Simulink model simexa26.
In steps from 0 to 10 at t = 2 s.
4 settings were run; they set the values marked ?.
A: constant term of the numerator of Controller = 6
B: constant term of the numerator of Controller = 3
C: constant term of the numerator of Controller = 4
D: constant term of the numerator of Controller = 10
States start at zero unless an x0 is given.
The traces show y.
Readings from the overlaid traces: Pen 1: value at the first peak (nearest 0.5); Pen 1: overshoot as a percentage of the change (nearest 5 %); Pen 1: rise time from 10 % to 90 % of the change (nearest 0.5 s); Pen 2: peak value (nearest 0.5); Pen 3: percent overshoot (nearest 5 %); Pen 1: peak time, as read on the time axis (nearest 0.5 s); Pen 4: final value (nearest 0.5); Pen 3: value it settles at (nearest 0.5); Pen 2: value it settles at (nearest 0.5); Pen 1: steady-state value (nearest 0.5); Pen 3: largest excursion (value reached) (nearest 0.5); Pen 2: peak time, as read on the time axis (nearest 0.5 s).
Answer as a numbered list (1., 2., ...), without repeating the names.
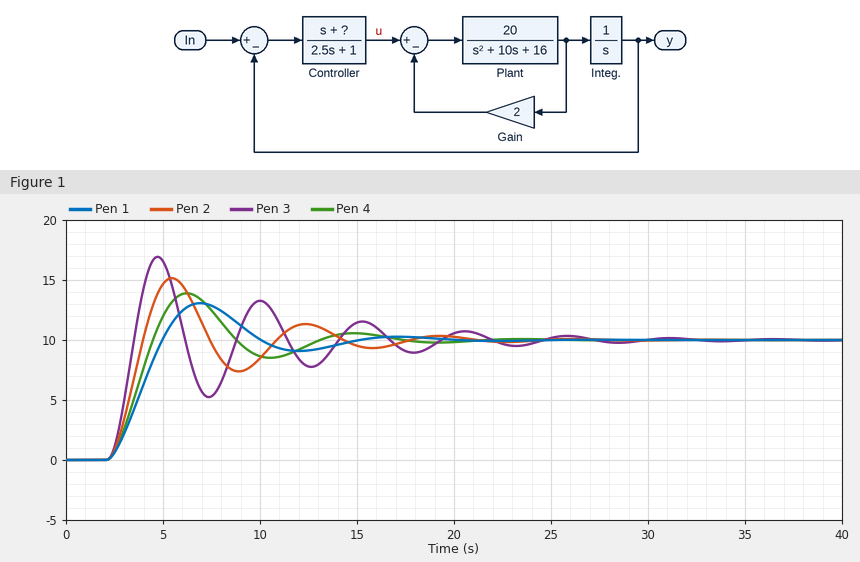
1. 13.0
2. 30 %
3. 2.0 s
4. 15.0
5. 70 %
6. 7.0 s
7. 10.0
8. 10.0
9. 10.0
10. 10.0
11. 17.0
12. 5.5 s
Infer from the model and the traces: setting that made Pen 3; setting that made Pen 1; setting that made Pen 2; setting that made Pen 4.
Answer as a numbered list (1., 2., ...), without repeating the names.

1. D
2. B
3. A
4. C
